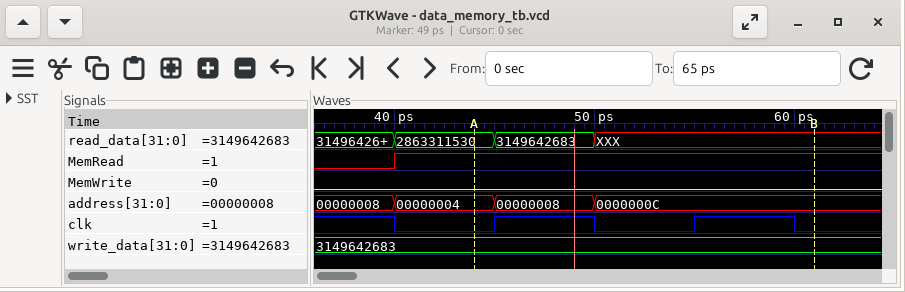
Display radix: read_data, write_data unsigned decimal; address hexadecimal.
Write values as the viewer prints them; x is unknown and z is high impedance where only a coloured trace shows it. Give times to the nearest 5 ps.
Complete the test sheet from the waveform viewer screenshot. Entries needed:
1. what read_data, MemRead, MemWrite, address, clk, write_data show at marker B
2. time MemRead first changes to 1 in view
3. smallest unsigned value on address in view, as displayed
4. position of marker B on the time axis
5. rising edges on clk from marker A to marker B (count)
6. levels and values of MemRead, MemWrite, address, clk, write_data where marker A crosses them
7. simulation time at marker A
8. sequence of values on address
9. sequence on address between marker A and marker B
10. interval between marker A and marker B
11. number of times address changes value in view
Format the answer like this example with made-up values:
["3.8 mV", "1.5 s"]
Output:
["read_data=XXX, MemRead=1, MemWrite=0, address=0000000C, clk=0, write_data=3149642683", "40 ps", "00000004", "60 ps", "2", "MemRead=1, MemWrite=0, address=00000004, clk=0, write_data=3149642683", "45 ps", "00000008, 00000004, 00000008, 0000000C", "00000004, 00000008, 0000000C", "15 ps", "3"]
